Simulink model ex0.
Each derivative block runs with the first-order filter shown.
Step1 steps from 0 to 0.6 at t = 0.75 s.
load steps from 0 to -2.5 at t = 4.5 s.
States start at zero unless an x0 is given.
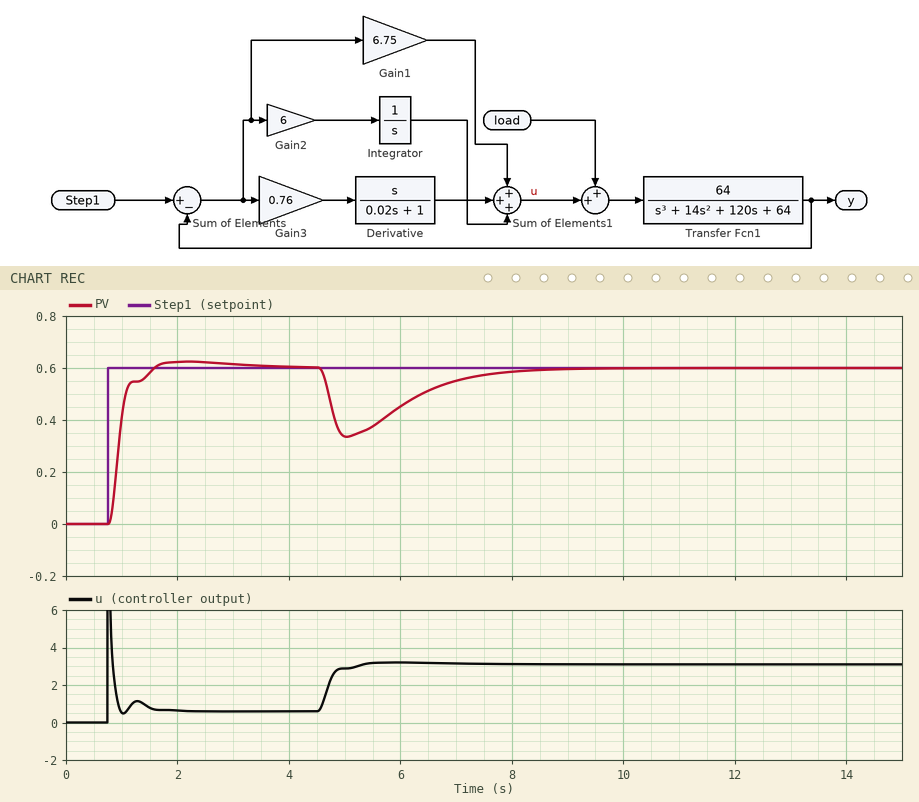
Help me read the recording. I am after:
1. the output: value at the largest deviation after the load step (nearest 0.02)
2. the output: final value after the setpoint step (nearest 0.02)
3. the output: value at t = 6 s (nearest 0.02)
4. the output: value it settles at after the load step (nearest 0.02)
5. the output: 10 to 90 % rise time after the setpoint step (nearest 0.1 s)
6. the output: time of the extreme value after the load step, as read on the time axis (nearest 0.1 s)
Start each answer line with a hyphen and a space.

- 0.34
- 0.60
- 0.46
- 0.60
- 0.3 s
- 5.0 s
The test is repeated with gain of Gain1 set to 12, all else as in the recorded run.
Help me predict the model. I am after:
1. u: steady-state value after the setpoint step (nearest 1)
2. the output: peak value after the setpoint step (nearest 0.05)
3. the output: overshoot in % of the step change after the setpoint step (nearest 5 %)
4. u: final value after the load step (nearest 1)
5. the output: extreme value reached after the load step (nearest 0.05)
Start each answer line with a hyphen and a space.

- 1
- 0.70
- 15 %
- 3
- 0.40
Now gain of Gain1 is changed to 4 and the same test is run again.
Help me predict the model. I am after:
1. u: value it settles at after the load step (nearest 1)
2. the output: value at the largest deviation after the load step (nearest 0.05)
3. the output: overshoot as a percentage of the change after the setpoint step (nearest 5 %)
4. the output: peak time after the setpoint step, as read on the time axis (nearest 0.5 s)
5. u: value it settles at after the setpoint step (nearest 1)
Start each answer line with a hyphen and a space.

- 3
- 0.25
- 10 %
- 2.5 s
- 1
